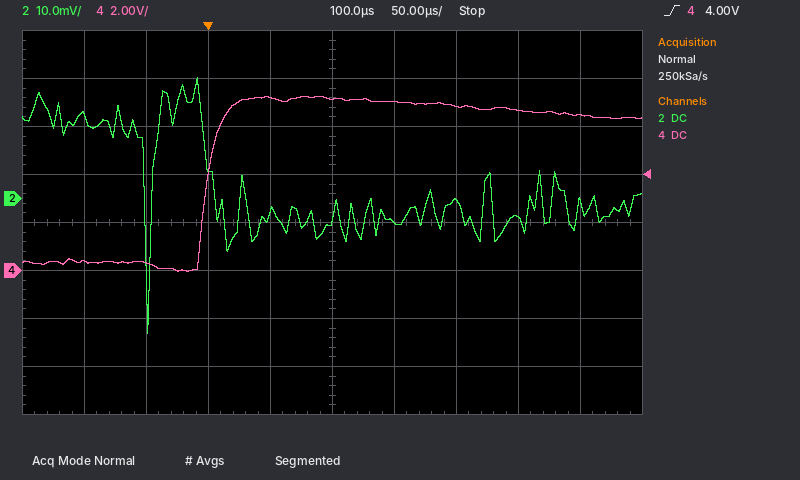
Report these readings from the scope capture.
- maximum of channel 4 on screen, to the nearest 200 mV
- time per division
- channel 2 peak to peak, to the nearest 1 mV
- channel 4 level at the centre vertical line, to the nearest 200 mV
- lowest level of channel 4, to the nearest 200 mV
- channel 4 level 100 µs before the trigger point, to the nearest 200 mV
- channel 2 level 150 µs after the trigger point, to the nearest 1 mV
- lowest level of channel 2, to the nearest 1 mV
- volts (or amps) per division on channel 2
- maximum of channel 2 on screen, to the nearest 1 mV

7.2 V
50 µs
53 mV
7.2 V
0.0 V
400 mV
-5 mV
-28 mV
10 mV
25 mV
